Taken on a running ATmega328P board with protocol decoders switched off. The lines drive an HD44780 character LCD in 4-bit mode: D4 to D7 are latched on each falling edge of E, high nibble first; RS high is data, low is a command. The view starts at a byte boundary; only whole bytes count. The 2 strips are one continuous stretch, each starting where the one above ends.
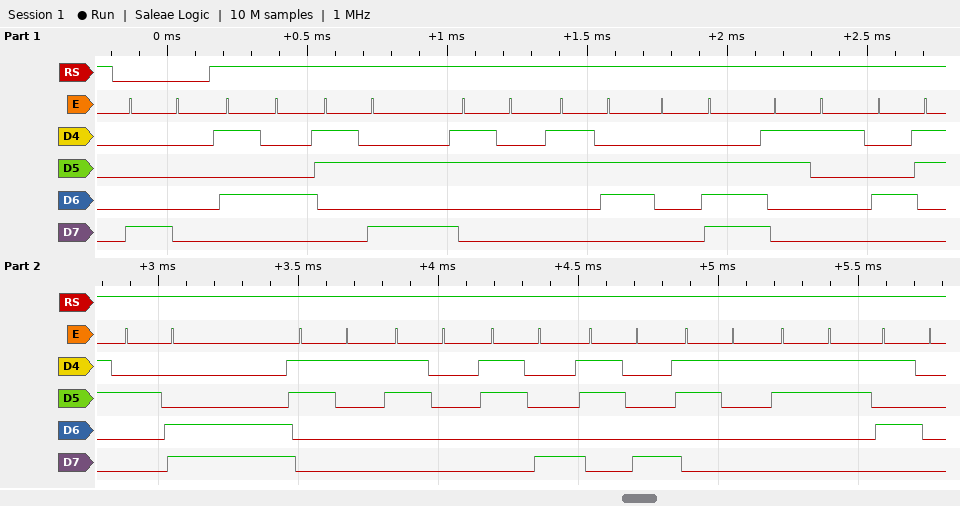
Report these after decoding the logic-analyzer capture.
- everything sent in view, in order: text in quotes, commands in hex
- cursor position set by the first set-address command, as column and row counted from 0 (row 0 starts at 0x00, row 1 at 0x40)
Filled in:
0x80 "T:26.1C,108813P"
column 0, row 0
